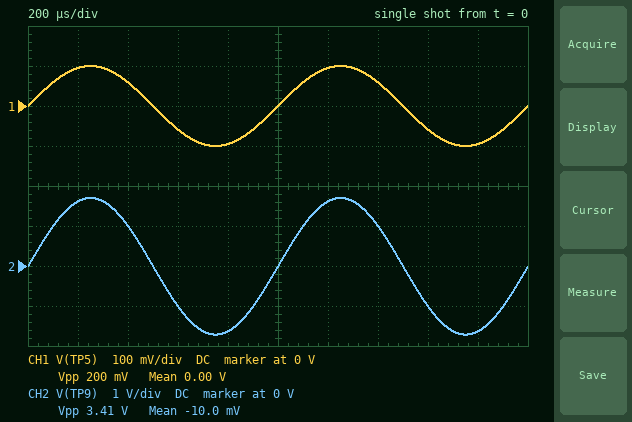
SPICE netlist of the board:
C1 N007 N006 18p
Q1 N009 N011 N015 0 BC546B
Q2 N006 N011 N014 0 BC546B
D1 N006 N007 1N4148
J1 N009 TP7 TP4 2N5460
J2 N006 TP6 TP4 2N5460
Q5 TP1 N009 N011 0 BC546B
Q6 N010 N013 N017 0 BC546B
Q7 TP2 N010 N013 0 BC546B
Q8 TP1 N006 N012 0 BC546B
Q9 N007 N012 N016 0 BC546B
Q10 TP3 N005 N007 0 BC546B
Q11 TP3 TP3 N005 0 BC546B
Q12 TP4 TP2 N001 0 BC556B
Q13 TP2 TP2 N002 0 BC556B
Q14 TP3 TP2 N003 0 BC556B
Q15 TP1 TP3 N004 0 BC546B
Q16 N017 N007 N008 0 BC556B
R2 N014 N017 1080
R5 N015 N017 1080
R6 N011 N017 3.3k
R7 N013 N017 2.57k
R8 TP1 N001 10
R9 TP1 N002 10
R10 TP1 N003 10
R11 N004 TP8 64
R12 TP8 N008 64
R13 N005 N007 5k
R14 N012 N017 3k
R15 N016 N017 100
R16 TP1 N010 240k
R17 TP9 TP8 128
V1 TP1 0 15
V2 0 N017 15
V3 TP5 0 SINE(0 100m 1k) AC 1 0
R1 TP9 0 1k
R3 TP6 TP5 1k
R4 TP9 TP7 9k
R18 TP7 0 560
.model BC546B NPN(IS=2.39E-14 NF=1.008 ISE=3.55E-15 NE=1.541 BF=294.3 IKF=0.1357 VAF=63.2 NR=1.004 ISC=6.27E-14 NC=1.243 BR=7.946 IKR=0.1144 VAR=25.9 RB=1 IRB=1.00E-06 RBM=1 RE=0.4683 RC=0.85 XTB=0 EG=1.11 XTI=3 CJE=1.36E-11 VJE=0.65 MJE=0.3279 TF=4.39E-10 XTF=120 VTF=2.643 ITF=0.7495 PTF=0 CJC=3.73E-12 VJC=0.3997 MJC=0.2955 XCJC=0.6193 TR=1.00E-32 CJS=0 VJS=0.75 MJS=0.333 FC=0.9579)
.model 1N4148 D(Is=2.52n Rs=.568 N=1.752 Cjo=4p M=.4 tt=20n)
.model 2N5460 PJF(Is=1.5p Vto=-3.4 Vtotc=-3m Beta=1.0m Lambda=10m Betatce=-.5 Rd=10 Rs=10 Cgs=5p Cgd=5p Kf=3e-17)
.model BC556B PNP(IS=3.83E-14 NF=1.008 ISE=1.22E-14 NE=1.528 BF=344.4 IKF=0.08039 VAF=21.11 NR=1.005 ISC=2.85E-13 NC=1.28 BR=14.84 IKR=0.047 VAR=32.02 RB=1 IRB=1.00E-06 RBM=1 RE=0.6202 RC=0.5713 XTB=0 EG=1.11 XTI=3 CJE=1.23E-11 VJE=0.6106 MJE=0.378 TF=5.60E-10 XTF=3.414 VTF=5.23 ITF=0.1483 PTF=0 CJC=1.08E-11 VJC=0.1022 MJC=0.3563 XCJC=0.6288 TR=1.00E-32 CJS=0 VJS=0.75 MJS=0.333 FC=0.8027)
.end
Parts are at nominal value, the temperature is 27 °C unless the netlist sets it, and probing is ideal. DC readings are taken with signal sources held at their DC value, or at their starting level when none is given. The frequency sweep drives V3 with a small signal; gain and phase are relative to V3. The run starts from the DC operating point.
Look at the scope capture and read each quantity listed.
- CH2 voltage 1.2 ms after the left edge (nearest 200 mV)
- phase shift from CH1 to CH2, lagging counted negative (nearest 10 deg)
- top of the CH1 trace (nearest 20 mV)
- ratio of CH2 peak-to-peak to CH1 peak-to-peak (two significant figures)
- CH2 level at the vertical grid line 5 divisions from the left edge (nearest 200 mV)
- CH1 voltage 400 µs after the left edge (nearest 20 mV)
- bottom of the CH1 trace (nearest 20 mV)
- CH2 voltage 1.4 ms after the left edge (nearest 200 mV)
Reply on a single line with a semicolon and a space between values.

1.6 V; 0 deg; 100 mV; 17; 0 V; 60 mV; -100 mV; 1.0 V
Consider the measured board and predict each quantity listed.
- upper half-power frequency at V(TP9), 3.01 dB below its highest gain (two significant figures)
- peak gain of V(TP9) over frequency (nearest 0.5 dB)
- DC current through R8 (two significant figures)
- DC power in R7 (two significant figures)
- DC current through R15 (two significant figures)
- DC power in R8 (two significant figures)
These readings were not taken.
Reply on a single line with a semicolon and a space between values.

360 kHz; 24.5 dB; 390 µA; 130 µW; 360 µA; 1.5 µW
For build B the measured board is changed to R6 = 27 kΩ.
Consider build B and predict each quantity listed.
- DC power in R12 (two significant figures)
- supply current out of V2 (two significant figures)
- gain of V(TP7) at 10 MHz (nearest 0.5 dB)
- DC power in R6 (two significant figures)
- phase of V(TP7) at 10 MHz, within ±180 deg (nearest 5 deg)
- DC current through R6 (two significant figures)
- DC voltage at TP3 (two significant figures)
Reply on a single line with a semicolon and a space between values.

2.3 µW; 1.5 mA; -25.0 dB; 24 µW; 85 deg; 30 µA; 610 mV
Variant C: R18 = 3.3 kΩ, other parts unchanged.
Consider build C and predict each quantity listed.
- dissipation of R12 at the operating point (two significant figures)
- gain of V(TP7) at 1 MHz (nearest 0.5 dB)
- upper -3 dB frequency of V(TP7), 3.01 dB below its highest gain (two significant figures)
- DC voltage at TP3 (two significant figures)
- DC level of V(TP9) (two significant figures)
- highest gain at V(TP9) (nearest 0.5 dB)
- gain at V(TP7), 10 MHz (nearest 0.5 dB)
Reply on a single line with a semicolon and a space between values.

2.4 µW; -1.0 dB; 1.9 MHz; 600 mV; -1.7 mV; 11.5 dB; -11.0 dB
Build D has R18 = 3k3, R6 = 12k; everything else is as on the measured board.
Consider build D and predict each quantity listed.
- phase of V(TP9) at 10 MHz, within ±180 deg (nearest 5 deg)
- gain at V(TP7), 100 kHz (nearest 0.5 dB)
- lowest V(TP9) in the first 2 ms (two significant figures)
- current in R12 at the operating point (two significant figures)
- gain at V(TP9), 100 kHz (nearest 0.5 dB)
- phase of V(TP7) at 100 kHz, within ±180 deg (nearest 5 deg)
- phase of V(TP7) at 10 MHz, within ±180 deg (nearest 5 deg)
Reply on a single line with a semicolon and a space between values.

170 deg; 0 dB; -370 mV; 190 µA; 11.5 dB; -5 deg; 70 deg
